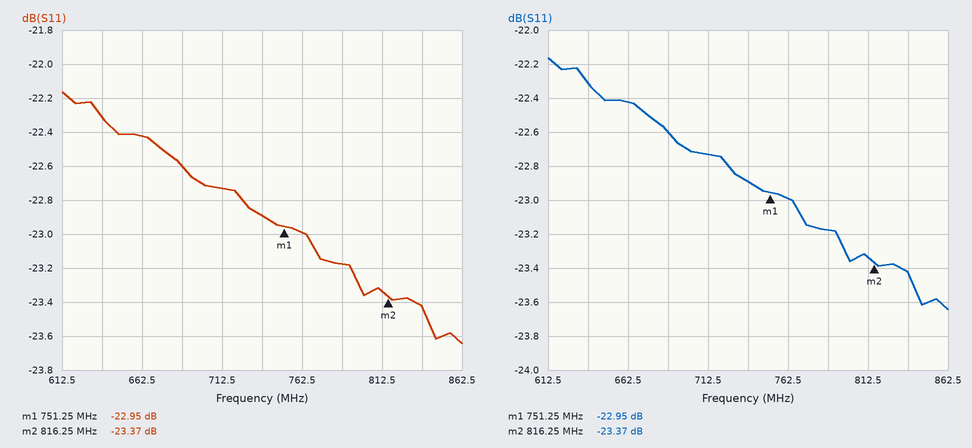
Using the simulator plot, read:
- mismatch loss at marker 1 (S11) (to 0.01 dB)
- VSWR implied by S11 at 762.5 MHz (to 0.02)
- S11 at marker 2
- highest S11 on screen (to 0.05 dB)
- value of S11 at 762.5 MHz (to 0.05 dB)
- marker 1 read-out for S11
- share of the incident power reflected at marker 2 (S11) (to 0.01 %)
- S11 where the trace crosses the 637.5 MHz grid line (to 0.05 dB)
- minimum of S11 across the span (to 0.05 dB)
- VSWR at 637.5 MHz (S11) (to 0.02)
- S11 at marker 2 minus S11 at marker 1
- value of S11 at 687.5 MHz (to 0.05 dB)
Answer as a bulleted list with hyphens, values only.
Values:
- 0.02 dB
- 1.16
- -23.37 dB
- -22.15 dB
- -23.00 dB
- -22.95 dB
- 0.46 %
- -22.30 dB
- -23.65 dB
- 1.16
- -0.42 dB
- -22.60 dB
